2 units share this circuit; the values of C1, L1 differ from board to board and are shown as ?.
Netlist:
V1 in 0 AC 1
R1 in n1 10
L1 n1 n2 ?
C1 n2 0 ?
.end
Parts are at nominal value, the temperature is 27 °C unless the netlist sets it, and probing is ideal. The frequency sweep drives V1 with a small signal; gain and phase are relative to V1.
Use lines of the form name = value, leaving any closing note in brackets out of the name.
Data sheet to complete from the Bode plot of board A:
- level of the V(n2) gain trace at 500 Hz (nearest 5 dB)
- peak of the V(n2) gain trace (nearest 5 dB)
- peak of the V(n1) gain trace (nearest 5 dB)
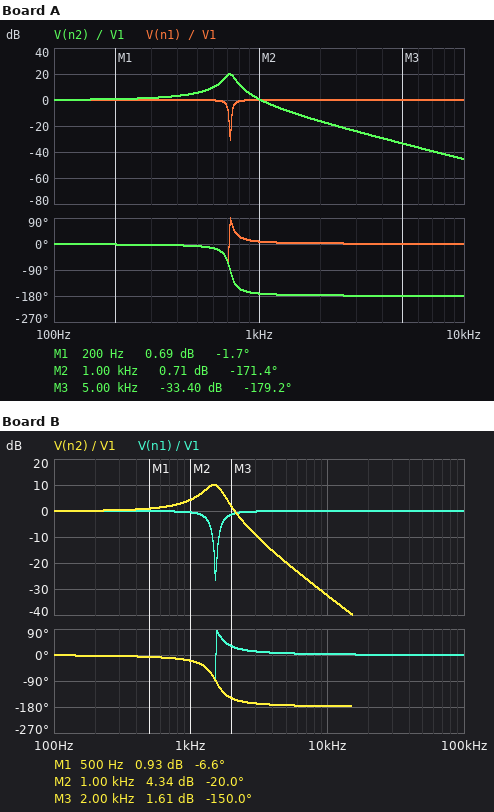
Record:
level of the V(n2) gain trace at 500 Hz = 5 dB
peak of the V(n2) gain trace = 20 dB
peak of the V(n1) gain trace = 0 dB
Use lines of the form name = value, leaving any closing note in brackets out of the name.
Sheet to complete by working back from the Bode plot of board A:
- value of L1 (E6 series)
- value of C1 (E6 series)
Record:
value of L1 = 22 mH
value of C1 = 2.2 µF
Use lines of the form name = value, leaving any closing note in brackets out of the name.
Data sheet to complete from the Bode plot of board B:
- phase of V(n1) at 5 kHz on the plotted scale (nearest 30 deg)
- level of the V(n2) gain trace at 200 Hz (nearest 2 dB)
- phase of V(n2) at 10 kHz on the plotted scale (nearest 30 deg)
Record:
phase of V(n1) at 5 kHz on the plotted scale = 0 deg
level of the V(n2) gain trace at 200 Hz = 0 dB
phase of V(n2) at 10 kHz on the plotted scale = -180 deg
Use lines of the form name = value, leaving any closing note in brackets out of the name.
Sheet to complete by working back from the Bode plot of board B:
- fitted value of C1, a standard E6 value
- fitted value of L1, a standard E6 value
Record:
fitted value of C1, a standard E6 value = 3.3 µF
fitted value of L1, a standard E6 value = 3.3 mH
